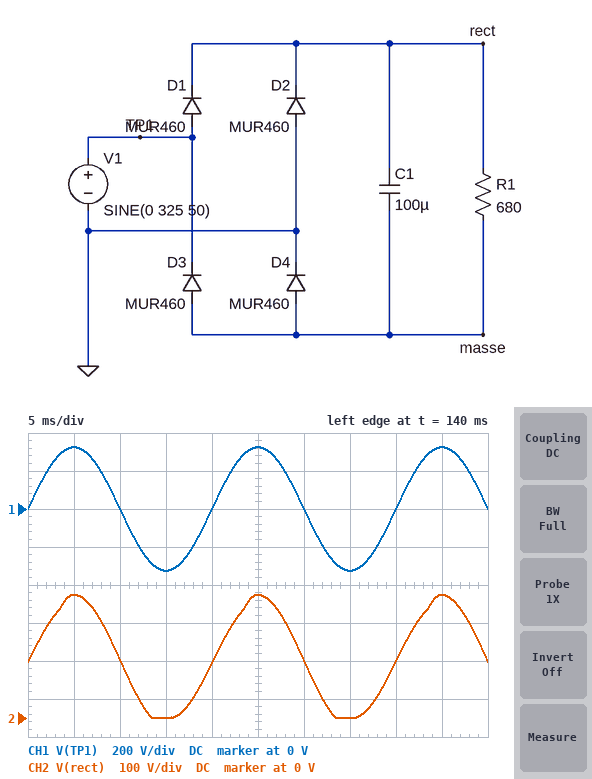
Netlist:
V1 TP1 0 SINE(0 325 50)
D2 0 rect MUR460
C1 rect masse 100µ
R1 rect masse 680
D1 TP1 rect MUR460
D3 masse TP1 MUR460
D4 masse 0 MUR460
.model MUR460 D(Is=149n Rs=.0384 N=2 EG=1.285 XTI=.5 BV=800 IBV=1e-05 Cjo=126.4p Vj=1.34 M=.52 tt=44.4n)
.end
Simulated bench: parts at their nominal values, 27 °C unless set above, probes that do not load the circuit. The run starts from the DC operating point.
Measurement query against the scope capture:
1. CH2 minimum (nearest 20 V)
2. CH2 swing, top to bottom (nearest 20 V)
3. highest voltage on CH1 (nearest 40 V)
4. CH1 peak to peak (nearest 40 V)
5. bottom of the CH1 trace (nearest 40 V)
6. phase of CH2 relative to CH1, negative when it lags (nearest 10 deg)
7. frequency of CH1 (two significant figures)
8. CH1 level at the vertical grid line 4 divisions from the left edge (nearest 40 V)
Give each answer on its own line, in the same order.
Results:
0 V
320 V
320 V
640 V
-320 V
0 deg
50 Hz
0 V
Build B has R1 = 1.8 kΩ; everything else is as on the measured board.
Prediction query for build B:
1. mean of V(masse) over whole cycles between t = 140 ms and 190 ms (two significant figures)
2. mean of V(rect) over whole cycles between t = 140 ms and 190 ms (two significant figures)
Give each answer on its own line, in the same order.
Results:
-160 V
160 V
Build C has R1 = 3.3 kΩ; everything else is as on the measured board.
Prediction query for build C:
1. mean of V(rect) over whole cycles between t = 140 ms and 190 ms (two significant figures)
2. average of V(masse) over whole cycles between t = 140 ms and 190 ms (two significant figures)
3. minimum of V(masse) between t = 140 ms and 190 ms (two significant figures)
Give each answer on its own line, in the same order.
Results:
160 V
-160 V
-320 V
